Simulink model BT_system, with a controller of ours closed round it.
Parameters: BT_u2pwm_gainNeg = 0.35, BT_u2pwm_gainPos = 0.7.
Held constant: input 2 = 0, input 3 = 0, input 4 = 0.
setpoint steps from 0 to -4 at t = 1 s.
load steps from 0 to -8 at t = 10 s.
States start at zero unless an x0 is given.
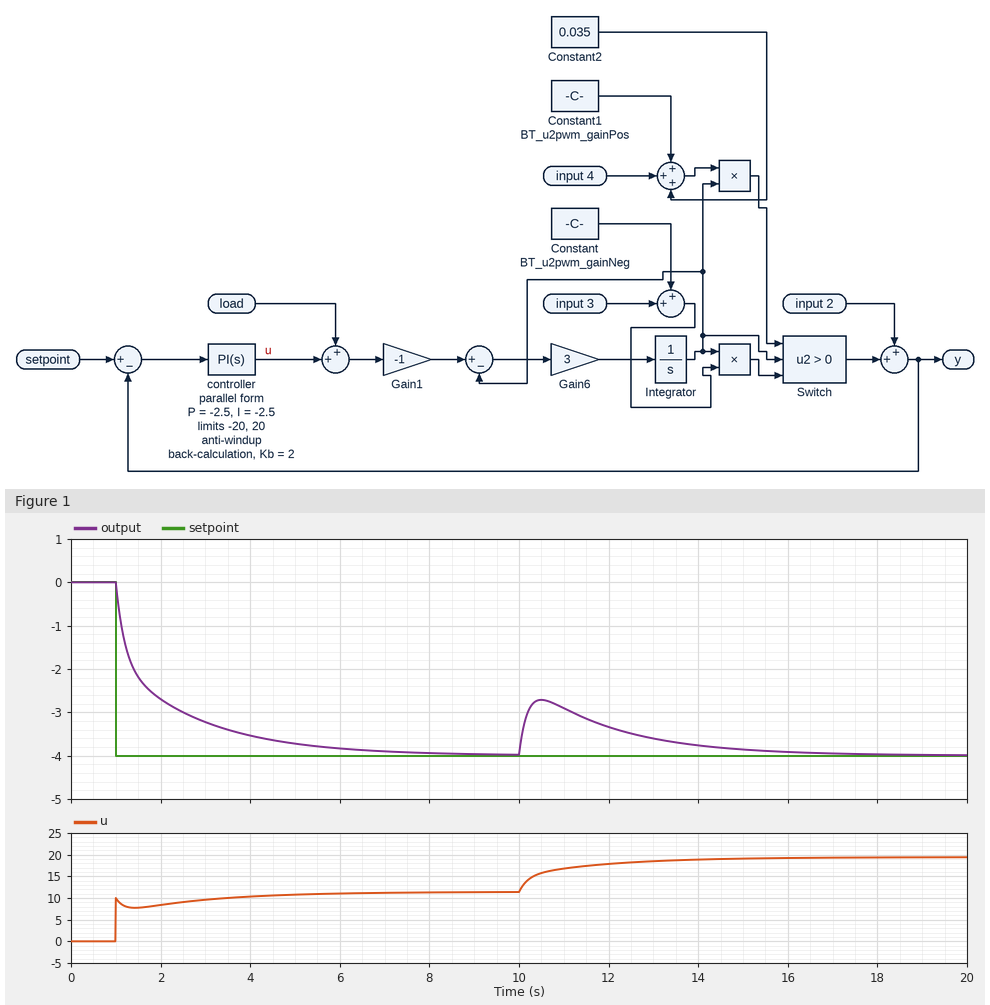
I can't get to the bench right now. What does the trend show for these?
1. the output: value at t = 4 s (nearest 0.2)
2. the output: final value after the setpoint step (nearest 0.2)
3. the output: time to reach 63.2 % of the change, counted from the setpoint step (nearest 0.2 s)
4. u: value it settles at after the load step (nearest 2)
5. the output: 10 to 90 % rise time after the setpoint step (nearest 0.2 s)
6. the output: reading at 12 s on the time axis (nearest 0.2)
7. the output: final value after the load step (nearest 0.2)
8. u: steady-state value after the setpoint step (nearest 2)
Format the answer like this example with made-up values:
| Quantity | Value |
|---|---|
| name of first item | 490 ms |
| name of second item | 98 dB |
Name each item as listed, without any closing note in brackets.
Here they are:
| Quantity | Value |
|---|---|
| the output: value at t = 4 s | -3.6 |
| the output: final value after the setpoint step | -4.0 |
| the output: time to reach 63.2 % of the change, counted from the setpoint step | 0.8 s |
| u: value it settles at after the load step | 20 |
| the output: 10 to 90 % rise time after the setpoint step | 3.2 s |
| the output: reading at 12 s on the time axis | -3.4 |
| the output: final value after the load step | -4.0 |
| u: steady-state value after the setpoint step | 12 |
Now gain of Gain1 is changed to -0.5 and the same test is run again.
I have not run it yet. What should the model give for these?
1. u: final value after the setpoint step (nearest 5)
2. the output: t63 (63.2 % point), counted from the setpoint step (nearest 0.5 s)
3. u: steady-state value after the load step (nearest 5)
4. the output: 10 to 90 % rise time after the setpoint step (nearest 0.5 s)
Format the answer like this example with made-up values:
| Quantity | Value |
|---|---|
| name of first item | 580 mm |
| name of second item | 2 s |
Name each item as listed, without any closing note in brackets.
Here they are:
| Quantity | Value |
|---|---|
| u: final value after the setpoint step | 20 |
| the output: t63 (63.2 % point), counted from the setpoint step | 1.5 s |
| u: steady-state value after the load step | 20 |
| the output: 10 to 90 % rise time after the setpoint step | 3.5 s |
